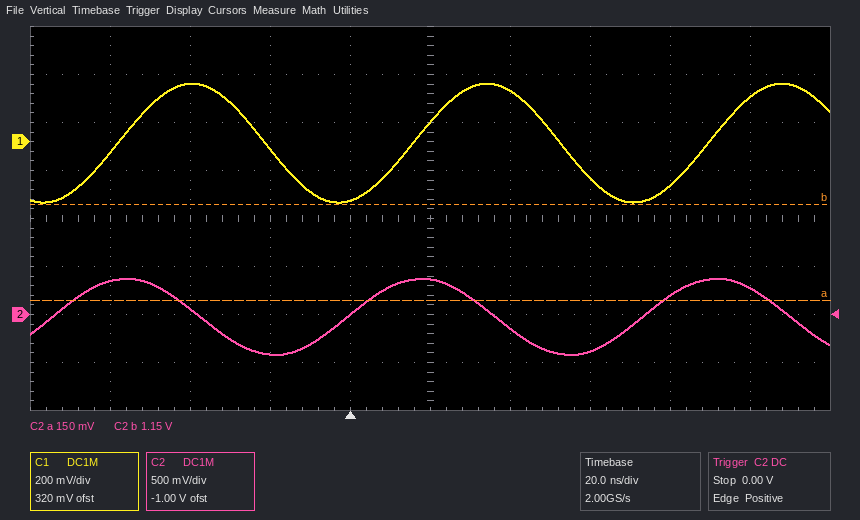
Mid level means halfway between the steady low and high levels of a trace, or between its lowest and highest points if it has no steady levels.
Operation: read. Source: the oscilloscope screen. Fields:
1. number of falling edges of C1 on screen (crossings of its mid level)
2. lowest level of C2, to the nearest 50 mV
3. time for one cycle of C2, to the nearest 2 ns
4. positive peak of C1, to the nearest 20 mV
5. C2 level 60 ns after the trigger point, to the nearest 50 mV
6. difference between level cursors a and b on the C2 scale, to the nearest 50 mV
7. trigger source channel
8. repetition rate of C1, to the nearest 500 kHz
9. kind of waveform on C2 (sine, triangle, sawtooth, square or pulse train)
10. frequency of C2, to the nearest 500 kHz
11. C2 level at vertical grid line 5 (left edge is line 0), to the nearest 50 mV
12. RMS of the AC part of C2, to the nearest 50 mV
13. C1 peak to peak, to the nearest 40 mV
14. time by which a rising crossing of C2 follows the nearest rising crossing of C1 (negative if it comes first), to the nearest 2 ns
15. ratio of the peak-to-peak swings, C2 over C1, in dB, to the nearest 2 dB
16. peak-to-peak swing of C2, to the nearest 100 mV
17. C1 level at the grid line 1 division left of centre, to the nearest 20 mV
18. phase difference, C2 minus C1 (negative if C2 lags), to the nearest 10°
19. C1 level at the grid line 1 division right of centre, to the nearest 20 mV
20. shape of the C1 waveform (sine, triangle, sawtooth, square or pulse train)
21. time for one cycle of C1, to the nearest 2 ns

2
-400 mV
74 ns
240 mV
-400 mV
1.00 V
C2
13.5 MHz
sine
13.5 MHz
350 mV
300 mV
480 mV
-16 ns
4 dB
800 mV
-240 mV
+80°
220 mV
sine
74 ns
